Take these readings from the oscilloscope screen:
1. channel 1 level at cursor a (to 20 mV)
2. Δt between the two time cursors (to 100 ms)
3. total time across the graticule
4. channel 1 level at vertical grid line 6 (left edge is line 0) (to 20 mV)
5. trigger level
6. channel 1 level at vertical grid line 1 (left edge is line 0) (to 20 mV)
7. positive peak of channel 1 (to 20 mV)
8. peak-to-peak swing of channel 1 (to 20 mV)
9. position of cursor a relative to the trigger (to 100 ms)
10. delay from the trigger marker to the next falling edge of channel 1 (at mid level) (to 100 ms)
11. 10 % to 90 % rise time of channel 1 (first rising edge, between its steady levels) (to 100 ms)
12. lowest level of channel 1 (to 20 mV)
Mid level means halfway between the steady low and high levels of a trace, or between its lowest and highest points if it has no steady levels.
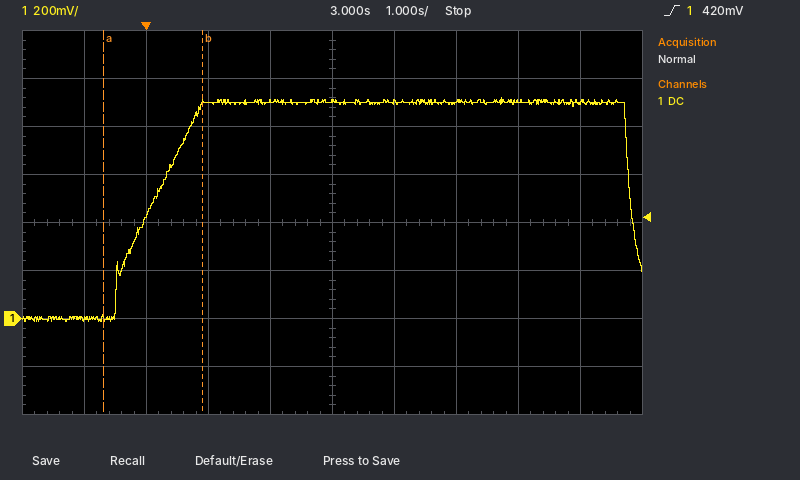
0 mV
1.6 s
10 s
900 mV
420 mV
0 mV
920 mV
940 mV
-700 ms
7.8 s
1.2 s
-20 mV
